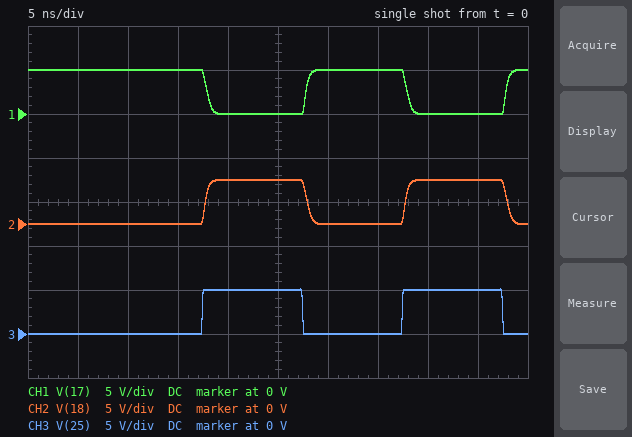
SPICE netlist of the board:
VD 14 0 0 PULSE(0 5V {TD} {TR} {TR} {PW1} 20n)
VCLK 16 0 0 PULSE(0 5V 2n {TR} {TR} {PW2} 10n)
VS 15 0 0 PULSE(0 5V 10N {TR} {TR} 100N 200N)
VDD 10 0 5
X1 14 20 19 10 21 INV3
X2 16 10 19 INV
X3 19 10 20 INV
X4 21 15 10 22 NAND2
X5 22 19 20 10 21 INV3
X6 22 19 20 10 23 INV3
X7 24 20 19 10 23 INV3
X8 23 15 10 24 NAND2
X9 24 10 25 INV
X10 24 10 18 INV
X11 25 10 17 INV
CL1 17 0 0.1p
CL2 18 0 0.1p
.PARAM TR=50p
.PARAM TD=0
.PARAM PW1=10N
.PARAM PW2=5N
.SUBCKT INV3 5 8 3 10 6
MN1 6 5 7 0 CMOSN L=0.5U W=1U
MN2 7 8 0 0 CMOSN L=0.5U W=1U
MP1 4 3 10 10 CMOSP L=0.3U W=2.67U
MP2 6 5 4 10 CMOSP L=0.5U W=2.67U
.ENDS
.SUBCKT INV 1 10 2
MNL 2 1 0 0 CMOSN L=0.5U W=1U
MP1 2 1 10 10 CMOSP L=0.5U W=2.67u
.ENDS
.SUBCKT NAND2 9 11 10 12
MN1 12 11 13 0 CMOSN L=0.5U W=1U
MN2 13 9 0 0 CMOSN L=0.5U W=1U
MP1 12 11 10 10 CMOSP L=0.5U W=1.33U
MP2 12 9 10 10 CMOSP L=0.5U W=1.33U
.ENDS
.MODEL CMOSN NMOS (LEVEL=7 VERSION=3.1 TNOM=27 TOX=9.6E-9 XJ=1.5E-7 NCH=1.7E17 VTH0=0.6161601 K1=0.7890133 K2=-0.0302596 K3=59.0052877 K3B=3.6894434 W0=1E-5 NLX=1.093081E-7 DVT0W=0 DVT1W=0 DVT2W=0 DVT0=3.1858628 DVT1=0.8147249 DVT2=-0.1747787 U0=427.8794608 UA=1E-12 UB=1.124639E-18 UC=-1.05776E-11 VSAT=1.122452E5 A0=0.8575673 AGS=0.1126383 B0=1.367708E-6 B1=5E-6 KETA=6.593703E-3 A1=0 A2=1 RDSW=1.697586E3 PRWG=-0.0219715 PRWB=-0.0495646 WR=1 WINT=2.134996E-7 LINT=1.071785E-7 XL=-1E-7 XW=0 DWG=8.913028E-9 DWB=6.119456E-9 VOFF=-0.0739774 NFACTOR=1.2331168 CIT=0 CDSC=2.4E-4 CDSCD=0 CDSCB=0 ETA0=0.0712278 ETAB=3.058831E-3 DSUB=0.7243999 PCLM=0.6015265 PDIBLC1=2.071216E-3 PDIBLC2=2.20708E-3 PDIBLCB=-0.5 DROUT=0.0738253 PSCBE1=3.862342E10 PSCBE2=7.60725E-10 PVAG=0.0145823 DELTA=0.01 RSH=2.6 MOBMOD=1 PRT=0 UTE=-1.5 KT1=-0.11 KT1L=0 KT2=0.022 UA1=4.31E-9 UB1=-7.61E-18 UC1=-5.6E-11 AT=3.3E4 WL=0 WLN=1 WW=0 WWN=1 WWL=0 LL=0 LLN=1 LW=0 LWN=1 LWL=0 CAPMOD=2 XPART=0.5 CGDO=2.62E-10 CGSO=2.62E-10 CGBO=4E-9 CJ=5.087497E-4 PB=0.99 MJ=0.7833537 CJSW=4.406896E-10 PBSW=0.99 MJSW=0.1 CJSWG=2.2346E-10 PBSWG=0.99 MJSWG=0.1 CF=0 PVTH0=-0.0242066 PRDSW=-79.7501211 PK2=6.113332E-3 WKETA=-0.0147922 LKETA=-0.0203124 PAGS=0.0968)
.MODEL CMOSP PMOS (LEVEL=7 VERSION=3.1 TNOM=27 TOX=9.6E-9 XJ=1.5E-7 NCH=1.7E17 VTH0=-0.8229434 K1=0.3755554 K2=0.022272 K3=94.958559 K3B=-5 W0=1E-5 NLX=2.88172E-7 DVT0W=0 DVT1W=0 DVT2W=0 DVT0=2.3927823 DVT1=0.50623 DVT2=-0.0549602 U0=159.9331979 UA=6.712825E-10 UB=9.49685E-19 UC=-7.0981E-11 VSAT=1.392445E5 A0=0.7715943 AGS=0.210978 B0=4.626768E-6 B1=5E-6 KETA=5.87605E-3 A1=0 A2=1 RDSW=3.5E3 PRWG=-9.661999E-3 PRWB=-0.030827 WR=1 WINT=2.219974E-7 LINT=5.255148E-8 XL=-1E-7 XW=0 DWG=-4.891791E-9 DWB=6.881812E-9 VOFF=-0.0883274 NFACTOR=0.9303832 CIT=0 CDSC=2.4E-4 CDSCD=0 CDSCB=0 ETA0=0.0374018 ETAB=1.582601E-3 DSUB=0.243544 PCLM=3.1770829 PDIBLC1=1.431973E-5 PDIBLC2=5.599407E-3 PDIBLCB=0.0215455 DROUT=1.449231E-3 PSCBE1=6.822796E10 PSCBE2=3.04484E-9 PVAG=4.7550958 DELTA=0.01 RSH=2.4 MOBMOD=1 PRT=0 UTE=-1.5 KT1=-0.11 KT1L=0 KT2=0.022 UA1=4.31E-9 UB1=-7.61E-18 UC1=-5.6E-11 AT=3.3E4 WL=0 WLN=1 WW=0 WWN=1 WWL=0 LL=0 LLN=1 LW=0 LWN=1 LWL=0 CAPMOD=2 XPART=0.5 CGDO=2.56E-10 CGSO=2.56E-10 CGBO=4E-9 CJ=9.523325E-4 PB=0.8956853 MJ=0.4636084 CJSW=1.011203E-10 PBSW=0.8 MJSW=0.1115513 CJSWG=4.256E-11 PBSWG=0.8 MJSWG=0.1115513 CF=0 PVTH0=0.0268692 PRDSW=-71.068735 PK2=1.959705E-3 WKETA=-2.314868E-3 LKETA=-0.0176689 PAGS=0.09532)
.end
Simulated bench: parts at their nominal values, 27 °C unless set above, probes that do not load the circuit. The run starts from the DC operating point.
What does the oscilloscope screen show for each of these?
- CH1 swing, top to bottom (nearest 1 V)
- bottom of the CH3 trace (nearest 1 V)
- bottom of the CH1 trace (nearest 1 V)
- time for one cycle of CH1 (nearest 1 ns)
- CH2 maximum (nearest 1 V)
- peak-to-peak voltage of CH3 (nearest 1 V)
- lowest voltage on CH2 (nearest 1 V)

5 V
0 V
0 V
20 ns
5 V
5 V
0 V
